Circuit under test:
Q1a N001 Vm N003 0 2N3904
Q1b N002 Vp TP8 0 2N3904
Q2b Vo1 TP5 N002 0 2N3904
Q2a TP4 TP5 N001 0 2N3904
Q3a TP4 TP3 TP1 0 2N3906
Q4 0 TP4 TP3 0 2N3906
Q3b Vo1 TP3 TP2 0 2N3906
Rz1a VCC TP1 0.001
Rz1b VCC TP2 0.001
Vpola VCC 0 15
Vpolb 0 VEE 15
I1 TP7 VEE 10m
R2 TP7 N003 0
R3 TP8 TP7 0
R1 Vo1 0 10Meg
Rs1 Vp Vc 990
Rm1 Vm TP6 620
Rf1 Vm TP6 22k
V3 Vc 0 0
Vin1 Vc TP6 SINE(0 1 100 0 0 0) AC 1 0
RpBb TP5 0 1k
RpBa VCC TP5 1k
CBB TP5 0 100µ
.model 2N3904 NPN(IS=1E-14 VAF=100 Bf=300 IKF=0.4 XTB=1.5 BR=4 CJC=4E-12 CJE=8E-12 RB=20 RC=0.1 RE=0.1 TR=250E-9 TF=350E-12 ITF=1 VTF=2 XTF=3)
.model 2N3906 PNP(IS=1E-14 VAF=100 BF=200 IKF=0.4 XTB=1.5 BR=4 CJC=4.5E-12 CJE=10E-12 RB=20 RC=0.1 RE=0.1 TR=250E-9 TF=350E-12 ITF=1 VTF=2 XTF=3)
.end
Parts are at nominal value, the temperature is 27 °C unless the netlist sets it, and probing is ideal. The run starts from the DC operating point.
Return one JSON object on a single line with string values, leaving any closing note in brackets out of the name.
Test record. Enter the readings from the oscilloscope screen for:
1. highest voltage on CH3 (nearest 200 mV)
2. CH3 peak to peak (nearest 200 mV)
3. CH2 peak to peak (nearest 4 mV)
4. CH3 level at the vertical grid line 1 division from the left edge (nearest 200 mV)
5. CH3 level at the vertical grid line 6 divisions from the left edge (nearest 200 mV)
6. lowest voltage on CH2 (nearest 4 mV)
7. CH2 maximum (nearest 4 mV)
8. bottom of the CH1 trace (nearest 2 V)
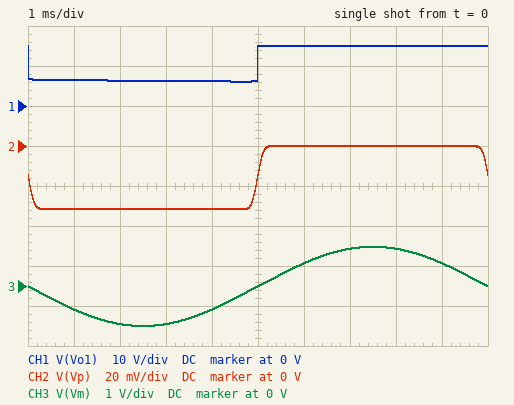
{"highest voltage on CH3": "1.0 V", "CH3 peak to peak": "2.0 V", "CH2 peak to peak": "32 mV", "CH3 level at the vertical grid line 1 division from the left edge": "-600 mV", "CH3 level at the vertical grid line 6 divisions from the left edge": "600 mV", "lowest voltage on CH2": "-32 mV", "CH2 maximum": "0 V", "bottom of the CH1 trace": "6 V"}
